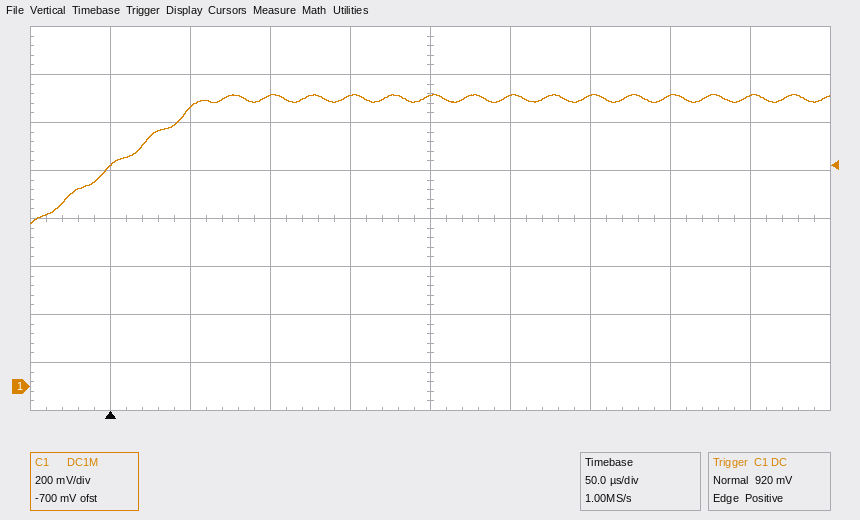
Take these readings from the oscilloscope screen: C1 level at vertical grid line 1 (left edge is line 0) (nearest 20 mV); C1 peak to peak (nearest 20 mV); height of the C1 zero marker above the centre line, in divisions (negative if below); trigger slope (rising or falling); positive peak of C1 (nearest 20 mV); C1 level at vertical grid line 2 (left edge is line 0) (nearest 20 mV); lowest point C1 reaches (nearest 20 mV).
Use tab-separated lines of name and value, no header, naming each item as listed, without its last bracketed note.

C1 level at vertical grid line 1 (left edge is line 0)	920 mV
C1 peak to peak	540 mV
height of the C1 zero marker above the centre line, in divisions	-3.5 div
trigger slope	rising
positive peak of C1	1.22 V
C1 level at vertical grid line 2 (left edge is line 0)	1.16 V
lowest point C1 reaches	680 mV
